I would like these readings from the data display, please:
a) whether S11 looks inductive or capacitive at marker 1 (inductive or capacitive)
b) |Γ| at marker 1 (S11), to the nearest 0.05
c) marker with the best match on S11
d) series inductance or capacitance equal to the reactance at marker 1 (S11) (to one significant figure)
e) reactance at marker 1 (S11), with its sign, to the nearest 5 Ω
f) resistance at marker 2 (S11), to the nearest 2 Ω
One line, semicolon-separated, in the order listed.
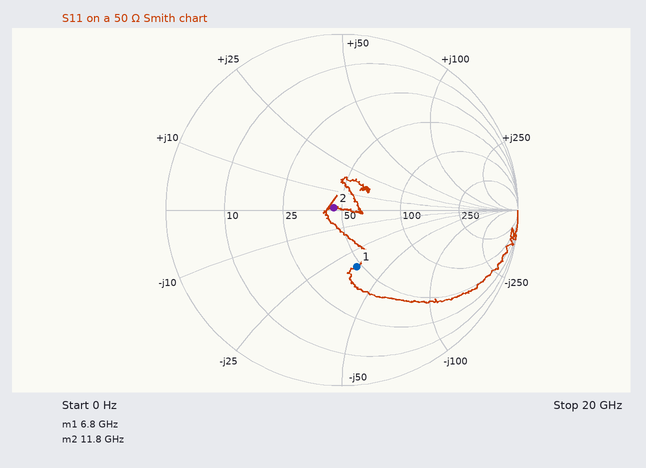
capacitive; 0.35; marker 2; 700 fF; -35 Ω; 46 Ω
